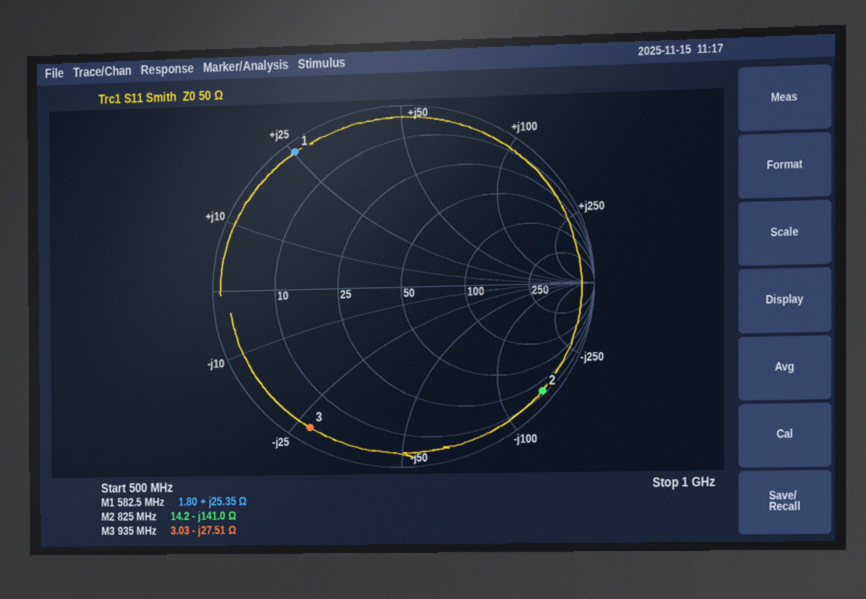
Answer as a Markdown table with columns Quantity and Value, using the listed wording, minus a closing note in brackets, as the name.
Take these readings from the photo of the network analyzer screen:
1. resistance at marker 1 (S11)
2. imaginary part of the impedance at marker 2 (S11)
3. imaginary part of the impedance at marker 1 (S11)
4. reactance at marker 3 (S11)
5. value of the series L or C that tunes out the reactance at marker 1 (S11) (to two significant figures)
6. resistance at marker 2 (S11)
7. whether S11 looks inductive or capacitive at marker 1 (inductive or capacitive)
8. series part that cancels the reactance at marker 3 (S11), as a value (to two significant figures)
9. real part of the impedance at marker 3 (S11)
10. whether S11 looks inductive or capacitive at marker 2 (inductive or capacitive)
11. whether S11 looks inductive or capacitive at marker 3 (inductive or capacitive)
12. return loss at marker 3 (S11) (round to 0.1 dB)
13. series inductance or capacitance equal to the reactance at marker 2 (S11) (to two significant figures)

| Quantity | Value |
|---|---|
| resistance at marker 1 | 1.80 Ω |
| imaginary part of the impedance at marker 2 | -141.0 Ω |
| imaginary part of the impedance at marker 1 | +25.35 Ω |
| reactance at marker 3 | -27.51 Ω |
| value of the series L or C that tunes out the reactance at marker 1 (S11) | 11 pF |
| resistance at marker 2 | 14.2 Ω |
| whether S11 looks inductive or capacitive at marker 1 | inductive |
| series part that cancels the reactance at marker 3 (S11), as a value | 4.7 nH |
| real part of the impedance at marker 3 | 3.03 Ω |
| whether S11 looks inductive or capacitive at marker 2 | capacitive |
| whether S11 looks inductive or capacitive at marker 3 | capacitive |
| return loss at marker 3 (S11) | 0.8 dB |
| series inductance or capacitance equal to the reactance at marker 2 (S11) | 1.4 pF |
